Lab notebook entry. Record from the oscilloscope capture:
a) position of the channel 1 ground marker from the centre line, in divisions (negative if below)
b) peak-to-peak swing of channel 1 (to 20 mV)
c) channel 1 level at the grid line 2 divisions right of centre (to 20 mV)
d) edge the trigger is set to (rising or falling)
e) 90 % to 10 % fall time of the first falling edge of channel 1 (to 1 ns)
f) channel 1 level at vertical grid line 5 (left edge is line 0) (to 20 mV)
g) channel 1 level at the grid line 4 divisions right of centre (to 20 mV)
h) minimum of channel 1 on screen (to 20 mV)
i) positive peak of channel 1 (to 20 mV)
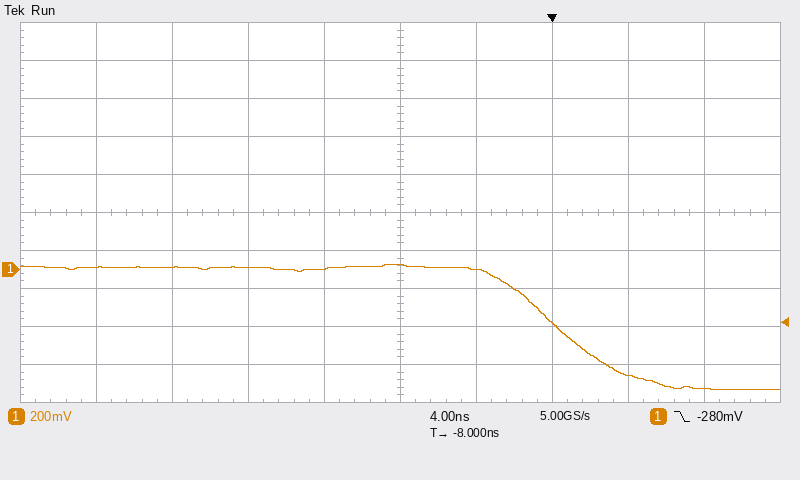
-1.5 div
660 mV
-280 mV
falling
7 ns
20 mV
-620 mV
-640 mV
20 mV
